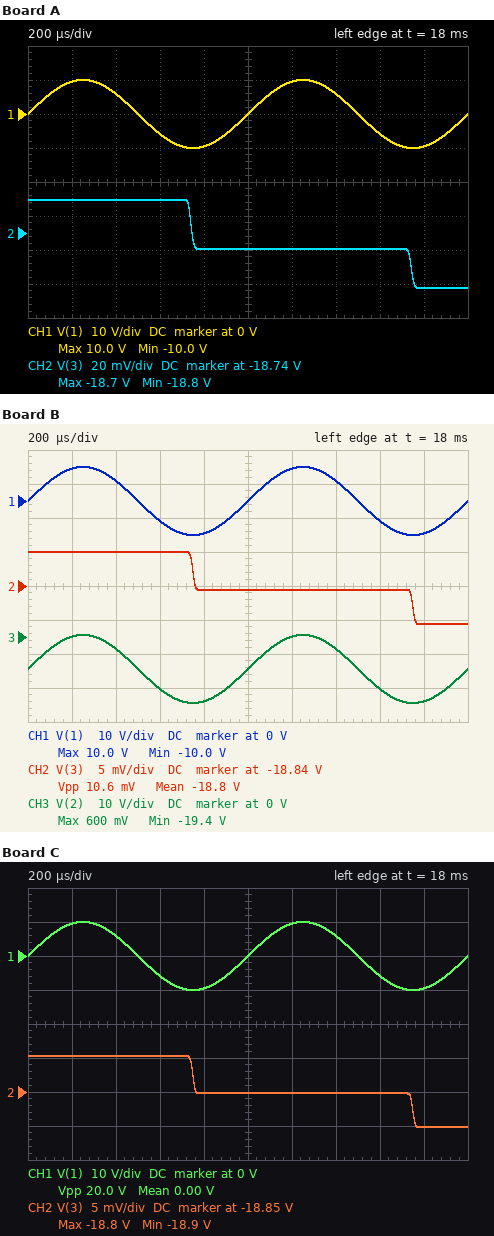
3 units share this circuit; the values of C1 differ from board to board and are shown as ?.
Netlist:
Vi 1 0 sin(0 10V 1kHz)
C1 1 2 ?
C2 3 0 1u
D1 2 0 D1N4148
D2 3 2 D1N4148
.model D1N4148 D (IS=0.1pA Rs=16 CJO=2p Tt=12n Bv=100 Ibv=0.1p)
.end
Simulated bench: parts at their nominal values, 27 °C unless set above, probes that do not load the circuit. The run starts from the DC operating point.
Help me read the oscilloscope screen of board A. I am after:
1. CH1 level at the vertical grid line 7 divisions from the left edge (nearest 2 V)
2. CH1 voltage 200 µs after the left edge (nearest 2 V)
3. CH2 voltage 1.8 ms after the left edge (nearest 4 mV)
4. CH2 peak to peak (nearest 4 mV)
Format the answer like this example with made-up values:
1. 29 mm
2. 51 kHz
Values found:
1. 6 V
2. 10 V
3. -18.772 V
4. 52 mV
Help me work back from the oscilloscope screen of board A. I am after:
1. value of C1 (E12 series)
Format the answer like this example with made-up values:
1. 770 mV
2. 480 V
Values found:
1. 330 nF
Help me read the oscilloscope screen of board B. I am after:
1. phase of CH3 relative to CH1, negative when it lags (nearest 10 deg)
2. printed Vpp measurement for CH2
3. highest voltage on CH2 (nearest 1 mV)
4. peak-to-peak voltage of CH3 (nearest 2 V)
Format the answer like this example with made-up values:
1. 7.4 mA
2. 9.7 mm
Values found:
1. 0 deg
2. 10.6 mV
3. -18.840 V
4. 20 V
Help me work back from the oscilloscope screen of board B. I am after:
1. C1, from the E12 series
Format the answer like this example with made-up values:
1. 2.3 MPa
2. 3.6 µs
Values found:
1. 2.7 µF
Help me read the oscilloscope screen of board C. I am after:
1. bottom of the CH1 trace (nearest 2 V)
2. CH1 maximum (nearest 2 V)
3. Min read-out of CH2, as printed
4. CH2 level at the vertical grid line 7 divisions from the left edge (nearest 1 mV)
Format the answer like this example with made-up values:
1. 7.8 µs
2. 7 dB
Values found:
1. -10 V
2. 10 V
3. -18.9 V
4. -18.850 V
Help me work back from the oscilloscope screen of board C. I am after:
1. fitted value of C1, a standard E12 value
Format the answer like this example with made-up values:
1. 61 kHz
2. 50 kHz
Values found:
1. 2.2 µF
